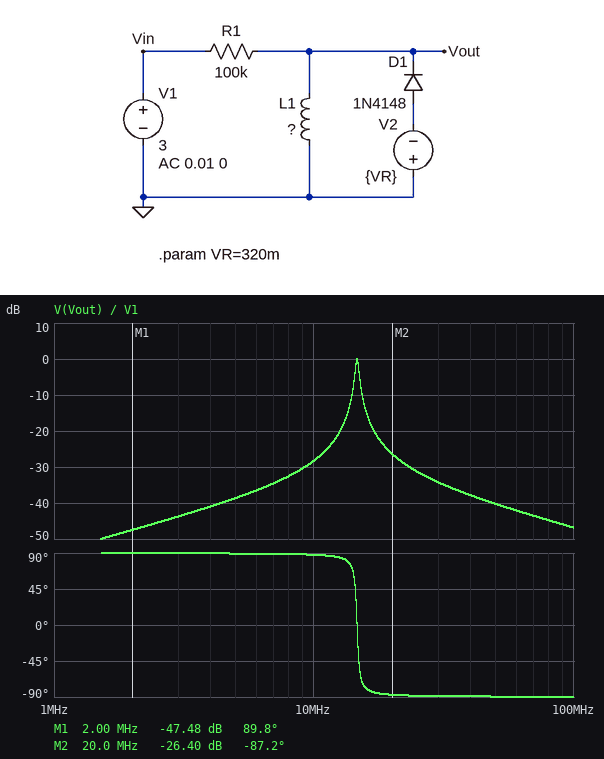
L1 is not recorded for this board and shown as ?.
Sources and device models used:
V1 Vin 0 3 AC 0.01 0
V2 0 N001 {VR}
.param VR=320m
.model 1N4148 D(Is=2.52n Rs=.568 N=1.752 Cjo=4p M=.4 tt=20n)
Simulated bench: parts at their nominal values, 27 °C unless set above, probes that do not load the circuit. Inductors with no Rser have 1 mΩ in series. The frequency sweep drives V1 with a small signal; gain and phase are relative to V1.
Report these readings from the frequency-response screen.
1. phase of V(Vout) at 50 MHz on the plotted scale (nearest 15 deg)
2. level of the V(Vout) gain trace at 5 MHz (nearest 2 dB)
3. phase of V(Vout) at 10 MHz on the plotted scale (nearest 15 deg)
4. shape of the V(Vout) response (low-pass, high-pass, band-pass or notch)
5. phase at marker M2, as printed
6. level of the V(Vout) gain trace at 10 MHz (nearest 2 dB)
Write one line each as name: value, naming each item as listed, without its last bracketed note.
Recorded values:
phase of V(Vout) at 50 MHz on the plotted scale: -90 deg
level of the V(Vout) gain trace at 5 MHz: -38 dB
phase of V(Vout) at 10 MHz on the plotted scale: 90 deg
shape of the V(Vout) response: band-pass
phase at marker M2, as printed: -87.2 deg
level of the V(Vout) gain trace at 10 MHz: -28 dB
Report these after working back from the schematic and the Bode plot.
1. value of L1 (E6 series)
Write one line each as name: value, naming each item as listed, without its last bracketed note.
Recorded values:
value of L1: 33 µH
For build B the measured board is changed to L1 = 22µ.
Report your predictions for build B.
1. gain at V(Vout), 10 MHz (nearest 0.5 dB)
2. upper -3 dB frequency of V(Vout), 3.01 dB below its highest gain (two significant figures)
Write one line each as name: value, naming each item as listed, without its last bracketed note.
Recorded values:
gain at V(Vout), 10 MHz: -34.0 dB
upper -3 dB frequency of V(Vout), 3.01 dB below its highest gain: 18 MHz
